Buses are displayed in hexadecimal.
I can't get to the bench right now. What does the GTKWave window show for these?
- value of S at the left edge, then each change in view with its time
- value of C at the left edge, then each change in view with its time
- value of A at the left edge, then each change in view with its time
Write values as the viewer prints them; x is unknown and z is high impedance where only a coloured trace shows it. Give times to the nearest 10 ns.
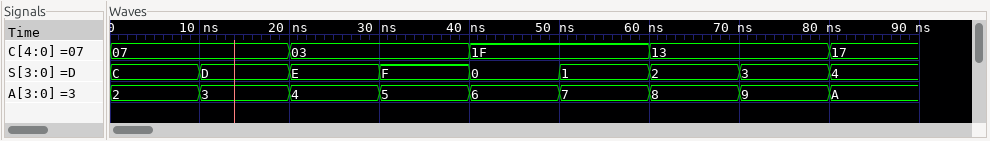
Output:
C, D at 10 ns, E at 20 ns, F at 30 ns, 0 at 40 ns, 1 at 50 ns, 2 at 60 ns, 3 at 70 ns, 4 at 80 ns
07, 03 at 20 ns, 1F at 40 ns, 13 at 60 ns, 17 at 80 ns
2, 3 at 10 ns, 4 at 20 ns, 5 at 30 ns, 6 at 40 ns, 7 at 50 ns, 8 at 60 ns, 9 at 70 ns, A at 80 ns
